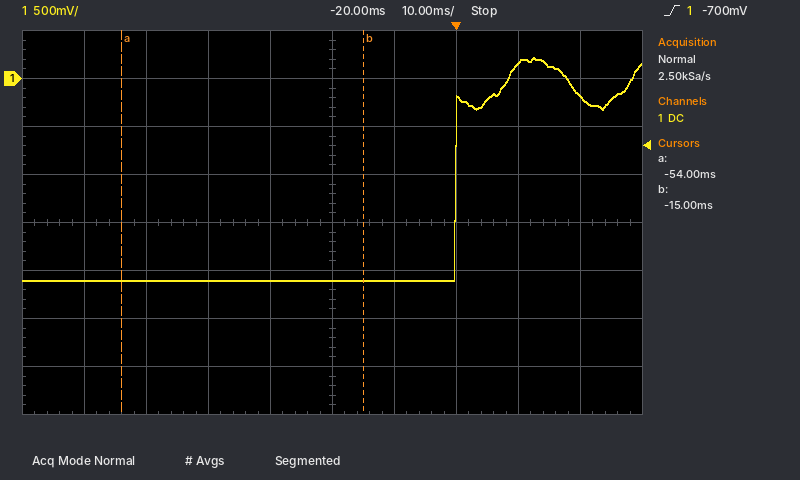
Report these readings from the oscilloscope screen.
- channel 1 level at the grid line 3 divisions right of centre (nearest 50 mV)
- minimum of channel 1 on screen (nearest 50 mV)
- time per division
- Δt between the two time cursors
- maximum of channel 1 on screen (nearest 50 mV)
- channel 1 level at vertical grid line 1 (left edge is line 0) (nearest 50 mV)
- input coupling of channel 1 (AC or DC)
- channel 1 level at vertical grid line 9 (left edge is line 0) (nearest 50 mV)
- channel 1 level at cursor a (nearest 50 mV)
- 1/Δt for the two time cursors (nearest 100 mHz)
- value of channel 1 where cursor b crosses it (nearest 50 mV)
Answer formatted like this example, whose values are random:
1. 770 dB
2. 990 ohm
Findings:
1. 150 mV
2. -2.10 V
3. 10 ms
4. 39 ms
5. 200 mV
6. -2.10 V
7. DC
8. -200 mV
9. -2.10 V
10. 25.6 Hz
11. -2.10 V
